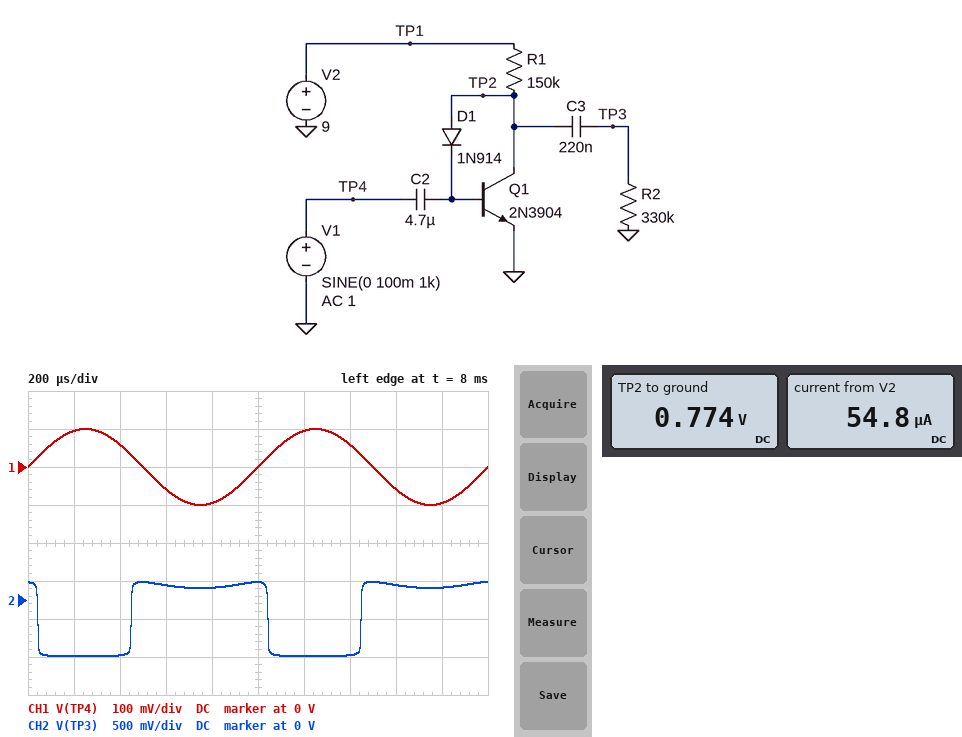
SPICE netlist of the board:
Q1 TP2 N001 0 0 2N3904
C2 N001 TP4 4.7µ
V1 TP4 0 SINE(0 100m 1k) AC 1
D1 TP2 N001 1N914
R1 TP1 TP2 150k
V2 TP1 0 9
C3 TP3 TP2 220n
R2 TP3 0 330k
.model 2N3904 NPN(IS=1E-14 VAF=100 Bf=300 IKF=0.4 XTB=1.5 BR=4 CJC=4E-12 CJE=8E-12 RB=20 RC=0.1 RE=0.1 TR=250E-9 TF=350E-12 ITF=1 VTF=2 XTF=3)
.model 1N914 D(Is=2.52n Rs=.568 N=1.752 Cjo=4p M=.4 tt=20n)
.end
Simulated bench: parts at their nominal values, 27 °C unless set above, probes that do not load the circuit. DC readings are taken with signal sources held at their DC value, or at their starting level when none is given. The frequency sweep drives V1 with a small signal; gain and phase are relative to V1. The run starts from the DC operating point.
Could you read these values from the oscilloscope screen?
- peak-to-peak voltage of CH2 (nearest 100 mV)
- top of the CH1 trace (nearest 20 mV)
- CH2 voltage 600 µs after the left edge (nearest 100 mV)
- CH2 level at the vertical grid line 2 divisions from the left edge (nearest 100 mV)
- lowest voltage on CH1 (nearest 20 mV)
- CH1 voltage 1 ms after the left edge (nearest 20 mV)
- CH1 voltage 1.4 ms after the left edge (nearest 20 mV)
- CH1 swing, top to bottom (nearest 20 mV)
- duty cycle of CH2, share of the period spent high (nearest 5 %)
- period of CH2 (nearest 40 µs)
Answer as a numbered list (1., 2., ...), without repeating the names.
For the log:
1. 1.0 V
2. 100 mV
3. 200 mV
4. -700 mV
5. -100 mV
6. 0 V
7. 60 mV
8. 200 mV
9. 60 %
10. 1.00 ms
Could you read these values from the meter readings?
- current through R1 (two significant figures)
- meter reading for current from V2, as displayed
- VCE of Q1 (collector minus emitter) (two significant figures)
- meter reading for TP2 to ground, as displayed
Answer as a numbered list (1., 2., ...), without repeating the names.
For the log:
1. 55 µA
2. 54.8 µA
3. 770 mV
4. 0.774 V
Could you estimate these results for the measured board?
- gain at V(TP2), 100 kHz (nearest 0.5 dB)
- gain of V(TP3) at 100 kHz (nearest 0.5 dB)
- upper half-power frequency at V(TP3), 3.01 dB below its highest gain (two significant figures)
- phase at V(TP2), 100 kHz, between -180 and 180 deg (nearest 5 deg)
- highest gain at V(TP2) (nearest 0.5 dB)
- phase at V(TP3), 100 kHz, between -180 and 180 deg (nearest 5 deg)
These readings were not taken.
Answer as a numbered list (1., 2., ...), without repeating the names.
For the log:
1. 43.0 dB
2. 43.0 dB
3. 270 kHz
4. 160 deg
5. 43.5 dB
6. 160 deg
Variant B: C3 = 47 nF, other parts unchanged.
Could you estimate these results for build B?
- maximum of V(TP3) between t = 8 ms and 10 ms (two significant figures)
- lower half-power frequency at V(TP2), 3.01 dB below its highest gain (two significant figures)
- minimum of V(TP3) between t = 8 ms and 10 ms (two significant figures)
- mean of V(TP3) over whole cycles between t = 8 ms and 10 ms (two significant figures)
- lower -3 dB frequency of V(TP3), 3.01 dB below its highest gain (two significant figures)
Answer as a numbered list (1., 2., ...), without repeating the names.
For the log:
1. 320 mV
2. 18 Hz
3. -670 mV
4. -110 mV
5. 22 Hz
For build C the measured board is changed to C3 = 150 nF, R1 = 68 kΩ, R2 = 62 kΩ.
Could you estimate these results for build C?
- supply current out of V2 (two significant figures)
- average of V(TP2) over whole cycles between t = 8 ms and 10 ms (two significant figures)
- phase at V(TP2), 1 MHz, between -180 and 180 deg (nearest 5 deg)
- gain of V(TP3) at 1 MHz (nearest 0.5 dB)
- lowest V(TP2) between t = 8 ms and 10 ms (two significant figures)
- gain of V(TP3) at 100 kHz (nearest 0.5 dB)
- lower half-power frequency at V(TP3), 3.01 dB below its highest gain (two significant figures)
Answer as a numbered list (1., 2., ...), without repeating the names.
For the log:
1. 120 µA
2. 600 mV
3. 125 deg
4. 36.5 dB
5. 8.4 mV
6. 41.0 dB
7. 34 Hz
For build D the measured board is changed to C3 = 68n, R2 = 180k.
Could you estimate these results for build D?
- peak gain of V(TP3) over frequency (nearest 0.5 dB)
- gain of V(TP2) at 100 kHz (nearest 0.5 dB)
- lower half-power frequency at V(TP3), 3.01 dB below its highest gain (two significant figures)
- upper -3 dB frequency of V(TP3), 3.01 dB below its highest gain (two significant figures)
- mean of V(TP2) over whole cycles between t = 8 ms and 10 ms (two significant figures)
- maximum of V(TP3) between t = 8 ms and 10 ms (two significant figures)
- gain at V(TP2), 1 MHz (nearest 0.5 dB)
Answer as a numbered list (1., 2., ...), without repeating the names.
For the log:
1. 42.0 dB
2. 41.5 dB
3. 19 Hz
4. 320 kHz
5. 570 mV
6. 340 mV
7. 31.5 dB
